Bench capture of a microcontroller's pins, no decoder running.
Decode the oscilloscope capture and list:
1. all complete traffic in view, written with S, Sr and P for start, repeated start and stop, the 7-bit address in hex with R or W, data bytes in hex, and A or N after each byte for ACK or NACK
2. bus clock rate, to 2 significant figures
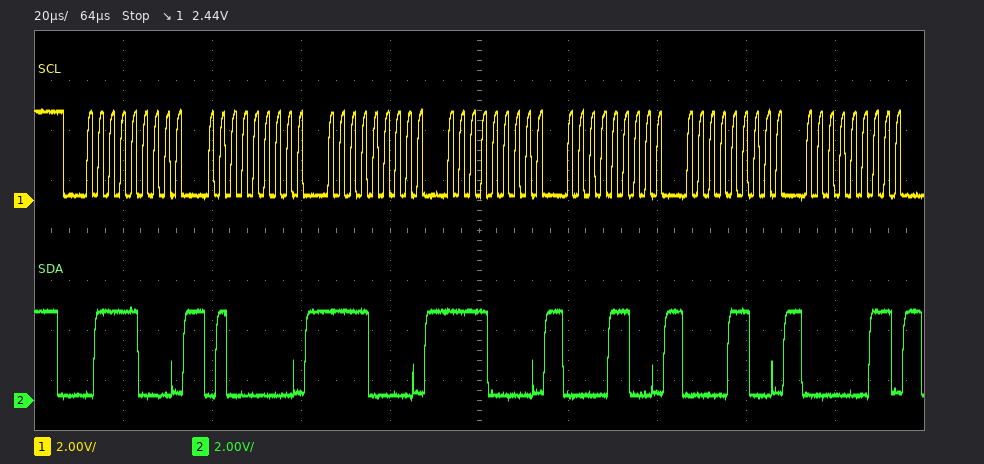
S 3CW A 40 A F0 A F0 A 0C A 0C A 03 A
400 kHz
